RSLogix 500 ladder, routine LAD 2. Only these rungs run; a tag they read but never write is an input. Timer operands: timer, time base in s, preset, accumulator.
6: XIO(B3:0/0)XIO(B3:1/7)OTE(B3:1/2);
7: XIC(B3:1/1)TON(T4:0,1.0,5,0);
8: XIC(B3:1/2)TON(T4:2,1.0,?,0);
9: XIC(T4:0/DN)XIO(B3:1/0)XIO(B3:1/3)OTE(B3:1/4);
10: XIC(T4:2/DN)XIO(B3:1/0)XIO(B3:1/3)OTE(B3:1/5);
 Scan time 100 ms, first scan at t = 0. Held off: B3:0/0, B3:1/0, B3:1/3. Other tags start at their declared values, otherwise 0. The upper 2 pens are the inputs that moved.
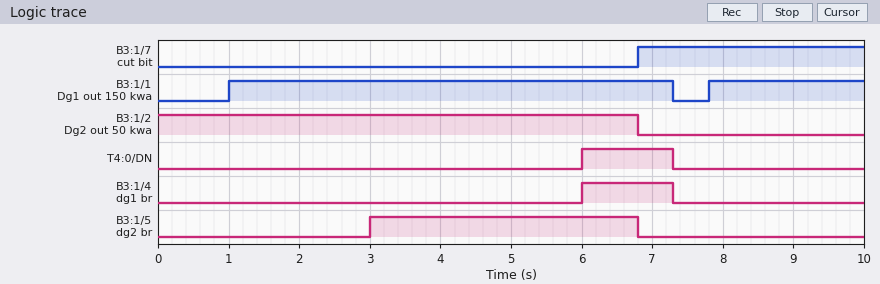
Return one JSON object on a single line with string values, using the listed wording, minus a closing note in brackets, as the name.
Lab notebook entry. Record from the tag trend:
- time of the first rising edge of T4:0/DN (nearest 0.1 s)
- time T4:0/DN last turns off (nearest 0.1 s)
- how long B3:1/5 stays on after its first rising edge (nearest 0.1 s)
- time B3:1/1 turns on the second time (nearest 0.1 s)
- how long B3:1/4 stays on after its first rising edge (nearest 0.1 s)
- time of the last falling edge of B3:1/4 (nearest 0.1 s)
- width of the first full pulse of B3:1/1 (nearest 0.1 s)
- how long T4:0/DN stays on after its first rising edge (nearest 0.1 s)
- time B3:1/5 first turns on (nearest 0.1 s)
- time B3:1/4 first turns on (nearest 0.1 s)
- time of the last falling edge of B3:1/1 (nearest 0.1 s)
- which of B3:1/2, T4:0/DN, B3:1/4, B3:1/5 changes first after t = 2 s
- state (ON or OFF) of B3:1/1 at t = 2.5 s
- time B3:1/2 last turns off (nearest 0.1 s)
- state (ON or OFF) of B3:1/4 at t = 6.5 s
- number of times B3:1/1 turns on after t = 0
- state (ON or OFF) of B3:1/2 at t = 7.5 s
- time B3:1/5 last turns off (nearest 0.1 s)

{"time of the first rising edge of T4:0/DN": "6.0 s", "time T4:0/DN last turns off": "7.3 s", "how long B3:1/5 stays on after its first rising edge": "3.8 s", "time B3:1/1 turns on the second time": "7.8 s", "how long B3:1/4 stays on after its first rising edge": "1.3 s", "time of the last falling edge of B3:1/4": "7.3 s", "width of the first full pulse of B3:1/1": "6.3 s", "how long T4:0/DN stays on after its first rising edge": "1.3 s", "time B3:1/5 first turns on": "3.0 s", "time B3:1/4 first turns on": "6.0 s", "time of the last falling edge of B3:1/1": "7.3 s", "which of B3:1/2, T4:0/DN, B3:1/4, B3:1/5 changes first after t = 2 s": "B3:1/5", "state (ON or OFF) of B3:1/1 at t = 2.5 s": "ON", "time B3:1/2 last turns off": "6.8 s", "state (ON or OFF) of B3:1/4 at t = 6.5 s": "ON", "number of times B3:1/1 turns on after t = 0": "2", "state (ON or OFF) of B3:1/2 at t = 7.5 s": "OFF", "time B3:1/5 last turns off": "6.8 s"}
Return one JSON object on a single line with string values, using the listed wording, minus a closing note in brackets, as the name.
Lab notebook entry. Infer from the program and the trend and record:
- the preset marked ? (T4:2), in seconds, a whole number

{"the preset marked ? (T4:2), in seconds, a whole number": "3 s"}
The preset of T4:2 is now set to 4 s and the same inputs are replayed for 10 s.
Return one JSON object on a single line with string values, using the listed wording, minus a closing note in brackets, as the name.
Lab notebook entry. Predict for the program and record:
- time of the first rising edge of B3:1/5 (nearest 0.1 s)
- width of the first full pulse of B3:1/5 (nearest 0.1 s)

{"time of the first rising edge of B3:1/5": "4.0 s", "width of the first full pulse of B3:1/5": "2.8 s"}
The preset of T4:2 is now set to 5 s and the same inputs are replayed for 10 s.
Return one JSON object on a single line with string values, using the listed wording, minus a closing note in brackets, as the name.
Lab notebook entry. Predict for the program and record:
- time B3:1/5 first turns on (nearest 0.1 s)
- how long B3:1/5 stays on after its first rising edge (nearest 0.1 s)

{"time B3:1/5 first turns on": "5.0 s", "how long B3:1/5 stays on after its first rising edge": "1.8 s"}
